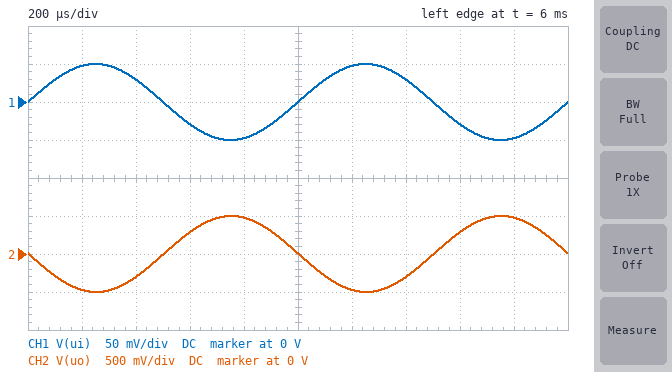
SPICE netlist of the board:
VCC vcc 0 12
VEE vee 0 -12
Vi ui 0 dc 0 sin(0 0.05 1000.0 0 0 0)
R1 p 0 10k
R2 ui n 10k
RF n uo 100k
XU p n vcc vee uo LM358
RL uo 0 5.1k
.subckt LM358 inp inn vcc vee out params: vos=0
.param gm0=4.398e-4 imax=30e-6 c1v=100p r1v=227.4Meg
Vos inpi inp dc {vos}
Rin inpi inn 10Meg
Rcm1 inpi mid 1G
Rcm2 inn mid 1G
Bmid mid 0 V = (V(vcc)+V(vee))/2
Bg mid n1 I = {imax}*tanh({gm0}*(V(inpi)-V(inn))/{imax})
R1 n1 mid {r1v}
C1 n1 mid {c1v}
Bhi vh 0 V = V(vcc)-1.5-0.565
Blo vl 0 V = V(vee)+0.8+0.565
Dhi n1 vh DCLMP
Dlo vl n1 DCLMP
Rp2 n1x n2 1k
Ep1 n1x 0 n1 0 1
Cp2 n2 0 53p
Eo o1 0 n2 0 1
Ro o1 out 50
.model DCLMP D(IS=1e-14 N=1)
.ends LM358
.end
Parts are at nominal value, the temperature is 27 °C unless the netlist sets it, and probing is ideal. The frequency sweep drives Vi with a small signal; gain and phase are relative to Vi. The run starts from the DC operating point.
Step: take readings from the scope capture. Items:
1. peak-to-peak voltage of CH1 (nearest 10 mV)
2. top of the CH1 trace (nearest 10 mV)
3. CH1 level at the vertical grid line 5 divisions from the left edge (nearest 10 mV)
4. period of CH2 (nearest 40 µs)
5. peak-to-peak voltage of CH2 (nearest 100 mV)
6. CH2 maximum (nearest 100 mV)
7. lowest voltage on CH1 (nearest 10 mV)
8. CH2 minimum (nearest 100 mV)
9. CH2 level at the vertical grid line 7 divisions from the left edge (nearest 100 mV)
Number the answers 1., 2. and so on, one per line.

1. 100 mV
2. 50 mV
3. 0 V
4. 1.00 ms
5. 1.0 V
6. 500 mV
7. -50 mV
8. -500 mV
9. -300 mV
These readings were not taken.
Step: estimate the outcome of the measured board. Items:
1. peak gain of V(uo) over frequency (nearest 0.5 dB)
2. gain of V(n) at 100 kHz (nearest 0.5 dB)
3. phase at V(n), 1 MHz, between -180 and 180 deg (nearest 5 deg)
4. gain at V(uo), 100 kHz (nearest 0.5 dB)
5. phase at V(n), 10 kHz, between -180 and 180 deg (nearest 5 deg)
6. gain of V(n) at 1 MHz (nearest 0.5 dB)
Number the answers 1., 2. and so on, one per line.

1. 20.0 dB
2. -2.0 dB
3. 5 deg
4. 14.5 dB
5. 80 deg
6. -0.5 dB
